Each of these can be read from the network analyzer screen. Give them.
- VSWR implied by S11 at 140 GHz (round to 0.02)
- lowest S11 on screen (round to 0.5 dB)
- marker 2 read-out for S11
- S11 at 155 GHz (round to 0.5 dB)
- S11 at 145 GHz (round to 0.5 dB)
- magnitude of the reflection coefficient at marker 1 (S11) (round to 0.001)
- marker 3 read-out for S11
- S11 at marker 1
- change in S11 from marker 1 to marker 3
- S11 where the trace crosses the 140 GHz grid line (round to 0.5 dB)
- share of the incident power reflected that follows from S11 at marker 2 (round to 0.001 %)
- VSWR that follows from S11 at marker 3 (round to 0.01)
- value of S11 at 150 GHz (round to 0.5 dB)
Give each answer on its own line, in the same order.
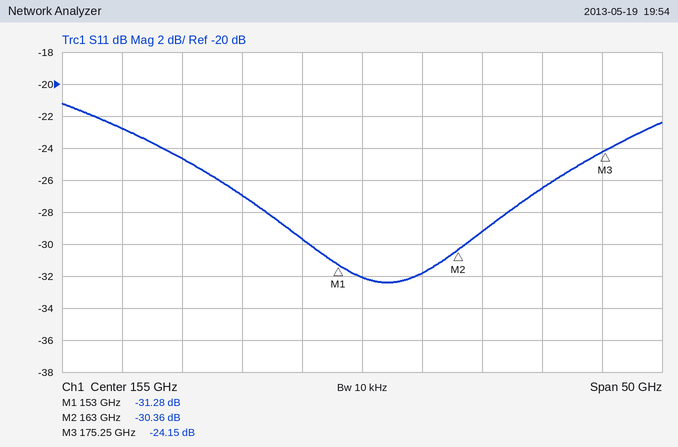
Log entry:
1.12
-32.5 dB
-30.36 dB
-32.0 dB
-27.0 dB
0.027
-24.15 dB
-31.28 dB
7.13 dB
-24.5 dB
0.092 %
1.13
-29.5 dB
